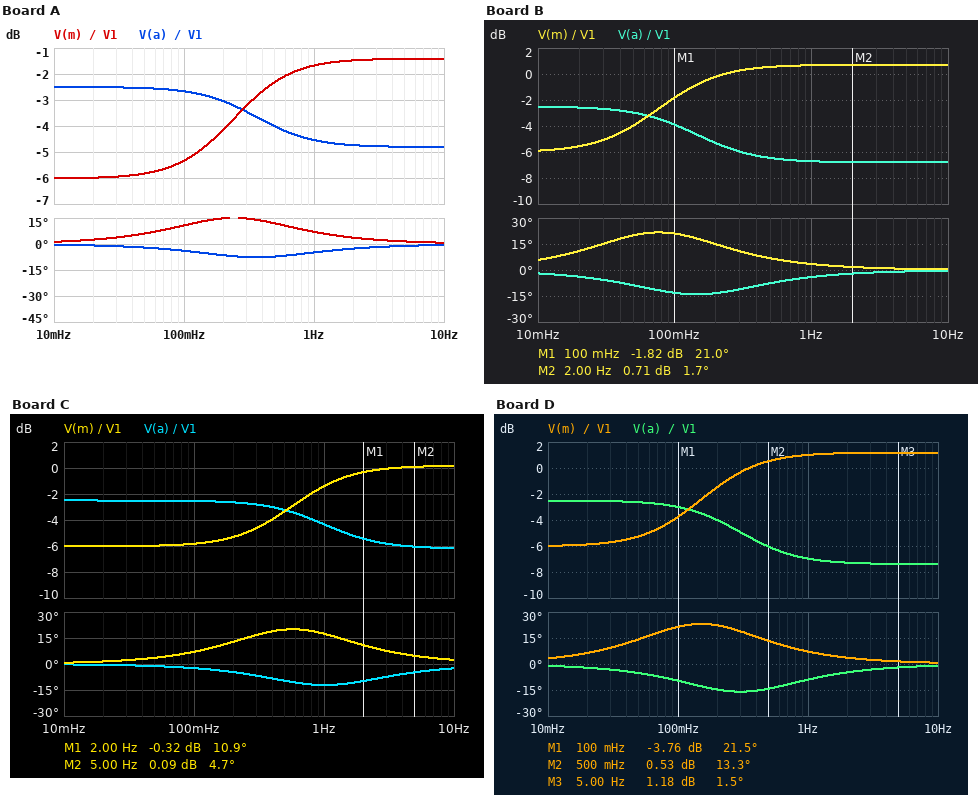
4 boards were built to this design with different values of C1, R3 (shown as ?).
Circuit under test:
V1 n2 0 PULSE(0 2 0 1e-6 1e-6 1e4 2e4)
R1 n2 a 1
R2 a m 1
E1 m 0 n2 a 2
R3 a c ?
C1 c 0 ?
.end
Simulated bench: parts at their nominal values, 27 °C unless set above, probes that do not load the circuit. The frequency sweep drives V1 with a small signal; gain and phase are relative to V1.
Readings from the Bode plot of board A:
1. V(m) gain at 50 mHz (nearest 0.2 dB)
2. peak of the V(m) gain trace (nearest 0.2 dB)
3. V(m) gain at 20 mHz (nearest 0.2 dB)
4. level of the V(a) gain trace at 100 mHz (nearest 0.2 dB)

-5.8 dB
-1.4 dB
-6.0 dB
-2.6 dB
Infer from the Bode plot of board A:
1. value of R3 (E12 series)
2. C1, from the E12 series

0.82 Ω
470 mF
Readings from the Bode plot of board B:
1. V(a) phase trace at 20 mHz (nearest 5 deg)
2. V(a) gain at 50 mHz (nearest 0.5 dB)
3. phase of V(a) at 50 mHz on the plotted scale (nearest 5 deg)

-5 deg
-3.0 dB
-10 deg
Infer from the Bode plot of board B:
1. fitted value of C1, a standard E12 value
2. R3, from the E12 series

2.2 F
0.39 Ω
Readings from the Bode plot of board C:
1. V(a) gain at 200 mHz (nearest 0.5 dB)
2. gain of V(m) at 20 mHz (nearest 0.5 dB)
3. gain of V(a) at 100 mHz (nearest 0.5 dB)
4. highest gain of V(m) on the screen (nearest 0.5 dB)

-2.5 dB
-6.0 dB
-2.5 dB
0 dB
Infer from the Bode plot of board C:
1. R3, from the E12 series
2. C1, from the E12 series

0.47 Ω
270 mF
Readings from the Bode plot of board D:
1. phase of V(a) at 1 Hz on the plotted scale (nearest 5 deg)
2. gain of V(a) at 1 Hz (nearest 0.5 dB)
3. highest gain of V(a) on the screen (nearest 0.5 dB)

-10 deg
-7.0 dB
-2.5 dB
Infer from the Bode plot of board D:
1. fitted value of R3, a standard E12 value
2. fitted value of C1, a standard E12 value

0.33 Ω
1.2 F
